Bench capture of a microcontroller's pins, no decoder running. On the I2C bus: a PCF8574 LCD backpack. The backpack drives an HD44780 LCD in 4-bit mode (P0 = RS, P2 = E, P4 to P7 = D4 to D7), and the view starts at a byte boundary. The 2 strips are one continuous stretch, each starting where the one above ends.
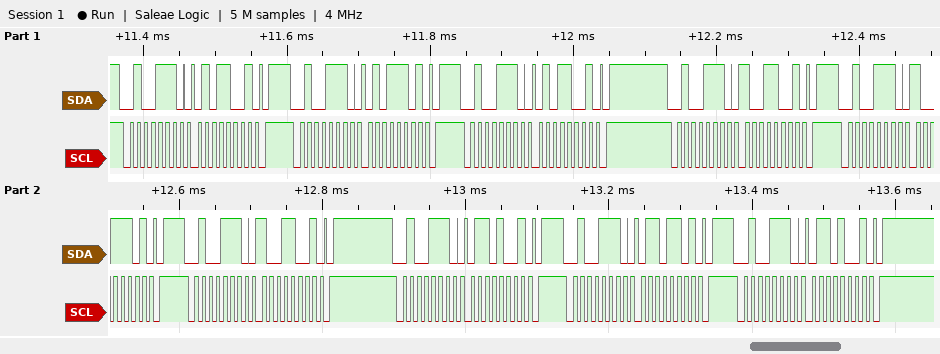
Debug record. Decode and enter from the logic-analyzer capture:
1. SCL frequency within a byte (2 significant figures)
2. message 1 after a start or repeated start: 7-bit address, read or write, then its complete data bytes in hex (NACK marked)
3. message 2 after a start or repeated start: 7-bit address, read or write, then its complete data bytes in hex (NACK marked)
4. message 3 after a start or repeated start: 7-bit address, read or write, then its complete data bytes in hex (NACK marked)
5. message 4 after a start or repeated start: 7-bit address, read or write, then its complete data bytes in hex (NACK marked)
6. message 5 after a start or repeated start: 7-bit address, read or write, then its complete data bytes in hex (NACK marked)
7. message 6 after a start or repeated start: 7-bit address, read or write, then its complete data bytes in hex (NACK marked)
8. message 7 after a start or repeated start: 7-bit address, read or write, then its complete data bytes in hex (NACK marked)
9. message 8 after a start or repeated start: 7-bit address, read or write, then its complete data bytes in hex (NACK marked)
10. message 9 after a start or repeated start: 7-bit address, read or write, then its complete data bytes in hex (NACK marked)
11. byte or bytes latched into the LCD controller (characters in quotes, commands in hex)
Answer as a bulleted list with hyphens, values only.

- 100 kHz
- 0x27 write: 59
- 0x27 write: 5D
- 0x27 write: 59
- 0x27 write: 99
- 0x27 write: 9D
- 0x27 write: 99
- 0x27 write: 69
- 0x27 write: 6D
- 0x27 write: 69
- 'Y'
